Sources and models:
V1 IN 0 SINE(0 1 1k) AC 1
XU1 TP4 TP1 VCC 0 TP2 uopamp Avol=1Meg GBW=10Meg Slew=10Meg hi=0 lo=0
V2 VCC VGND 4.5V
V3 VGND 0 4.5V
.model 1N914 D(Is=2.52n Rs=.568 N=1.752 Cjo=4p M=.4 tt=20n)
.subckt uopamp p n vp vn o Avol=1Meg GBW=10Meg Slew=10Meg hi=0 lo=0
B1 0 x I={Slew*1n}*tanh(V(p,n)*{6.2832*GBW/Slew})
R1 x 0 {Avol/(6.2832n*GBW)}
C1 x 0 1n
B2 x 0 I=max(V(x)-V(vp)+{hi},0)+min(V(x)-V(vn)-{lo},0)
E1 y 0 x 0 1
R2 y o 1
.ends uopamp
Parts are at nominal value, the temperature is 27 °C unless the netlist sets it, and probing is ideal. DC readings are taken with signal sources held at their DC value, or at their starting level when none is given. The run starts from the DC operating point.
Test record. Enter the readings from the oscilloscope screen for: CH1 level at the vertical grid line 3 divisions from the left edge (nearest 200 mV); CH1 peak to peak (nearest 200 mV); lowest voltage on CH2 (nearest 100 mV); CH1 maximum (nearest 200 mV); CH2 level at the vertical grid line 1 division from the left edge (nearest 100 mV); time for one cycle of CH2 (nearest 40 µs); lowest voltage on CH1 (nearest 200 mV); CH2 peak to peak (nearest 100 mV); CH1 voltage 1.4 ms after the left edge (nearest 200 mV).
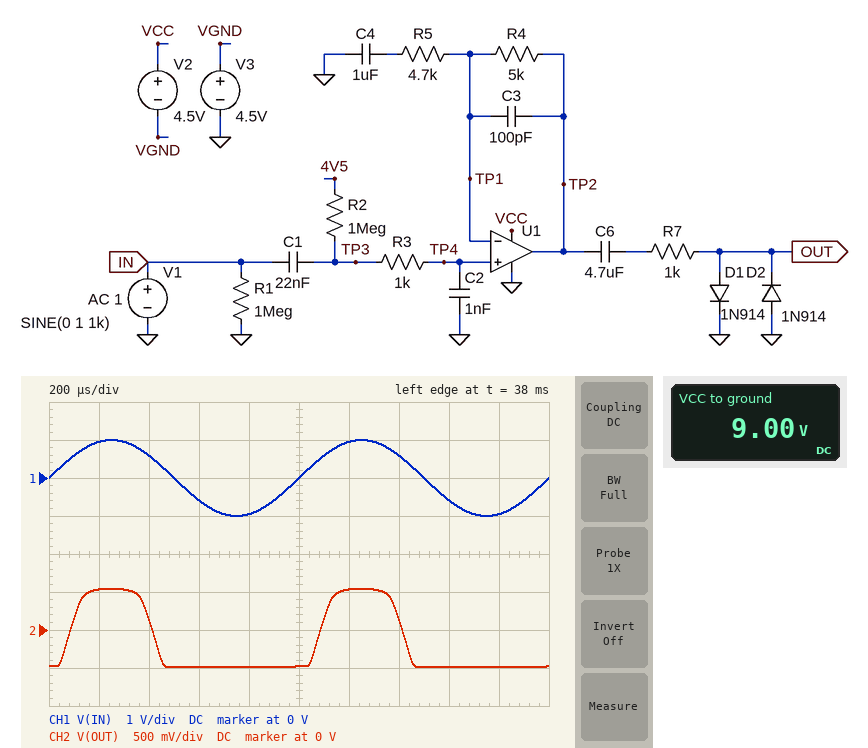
-600 mV
2.0 V
-500 mV
1.0 V
500 mV
1.00 ms
-1.0 V
1.0 V
600 mV
